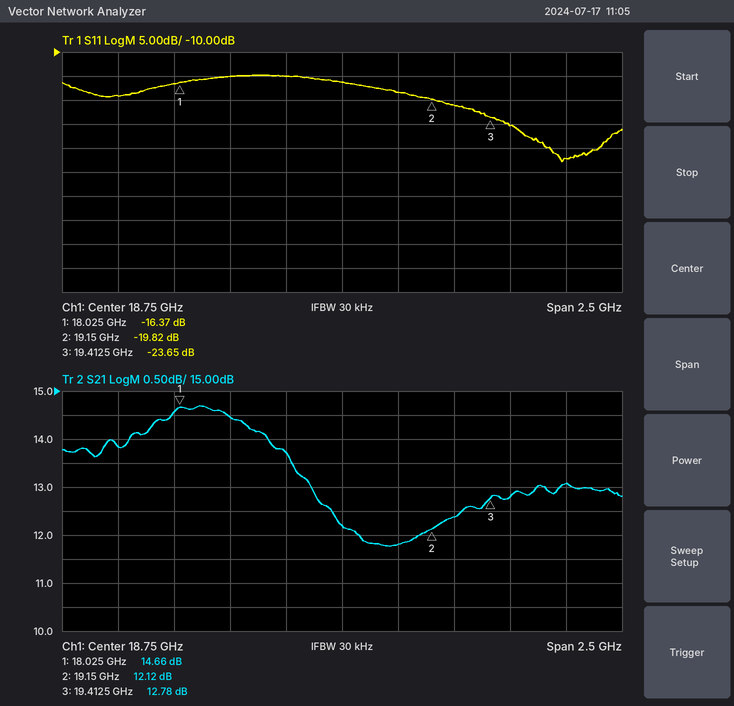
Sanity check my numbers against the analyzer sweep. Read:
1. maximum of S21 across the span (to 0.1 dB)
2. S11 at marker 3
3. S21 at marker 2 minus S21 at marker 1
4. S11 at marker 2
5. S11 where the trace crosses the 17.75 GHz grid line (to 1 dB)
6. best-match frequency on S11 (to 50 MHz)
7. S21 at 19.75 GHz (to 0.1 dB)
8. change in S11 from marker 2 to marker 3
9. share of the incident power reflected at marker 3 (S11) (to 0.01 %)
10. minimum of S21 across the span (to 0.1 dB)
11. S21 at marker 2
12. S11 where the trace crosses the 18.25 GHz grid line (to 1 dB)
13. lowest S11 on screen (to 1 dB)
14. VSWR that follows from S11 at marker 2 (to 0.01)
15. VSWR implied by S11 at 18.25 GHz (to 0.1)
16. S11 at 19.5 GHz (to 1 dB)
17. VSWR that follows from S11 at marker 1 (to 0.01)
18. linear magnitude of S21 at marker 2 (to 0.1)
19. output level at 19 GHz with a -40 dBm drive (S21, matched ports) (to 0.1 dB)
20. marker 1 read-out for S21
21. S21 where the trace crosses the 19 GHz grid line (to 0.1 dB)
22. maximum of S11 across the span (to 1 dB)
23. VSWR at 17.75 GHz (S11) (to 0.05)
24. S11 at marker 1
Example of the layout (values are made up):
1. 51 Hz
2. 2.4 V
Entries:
1. 14.7 dB
2. -23.65 dB
3. -2.54 dB
4. -19.82 dB
5. -19 dB
6. 19.75 GHz
7. 13.1 dB
8. -3.83 dB
9. 0.43 %
10. 11.8 dB
11. 12.12 dB
12. -15 dB
13. -33 dB
14. 1.23
15. 1.4
16. -25 dB
17. 1.36
18. 4.0
19. -28.2 dBm
20. 14.66 dB
21. 11.8 dB
22. -15 dB
23. 1.25
24. -16.37 dB
